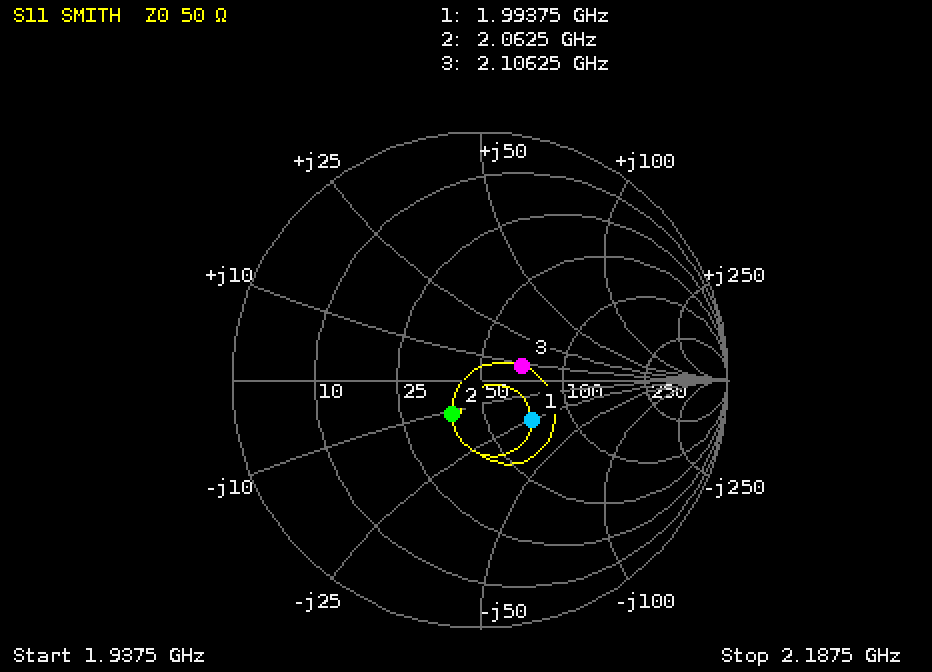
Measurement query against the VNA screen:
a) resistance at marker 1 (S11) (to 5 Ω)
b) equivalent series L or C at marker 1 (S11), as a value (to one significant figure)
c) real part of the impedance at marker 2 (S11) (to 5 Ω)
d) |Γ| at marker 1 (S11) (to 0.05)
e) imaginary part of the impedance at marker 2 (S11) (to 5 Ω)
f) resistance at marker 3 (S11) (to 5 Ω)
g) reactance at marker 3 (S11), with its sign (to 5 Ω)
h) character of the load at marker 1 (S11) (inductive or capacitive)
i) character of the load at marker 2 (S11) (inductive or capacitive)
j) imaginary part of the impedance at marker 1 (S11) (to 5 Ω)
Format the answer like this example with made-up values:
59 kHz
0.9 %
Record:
70 Ω
3 pF
40 Ω
0.25
-10 Ω
70 Ω
+10 Ω
capacitive
capacitive
-25 Ω
